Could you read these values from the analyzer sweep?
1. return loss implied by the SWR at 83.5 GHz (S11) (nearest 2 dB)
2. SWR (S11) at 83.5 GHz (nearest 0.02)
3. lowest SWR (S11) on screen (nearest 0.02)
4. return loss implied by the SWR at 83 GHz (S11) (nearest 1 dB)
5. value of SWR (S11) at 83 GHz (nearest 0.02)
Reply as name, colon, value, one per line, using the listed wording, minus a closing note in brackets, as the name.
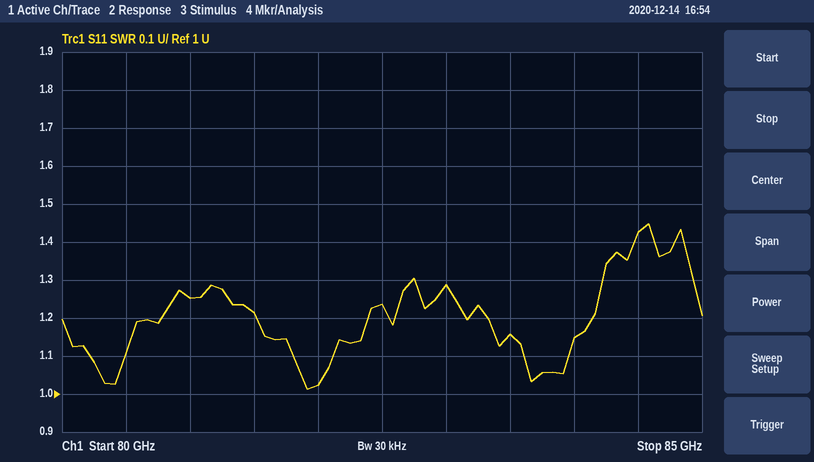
return loss implied by the SWR at 83.5 GHz (S11): 22 dB
SWR (S11) at 83.5 GHz: 1.16
lowest SWR (S11) on screen: 1.02
return loss implied by the SWR at 83 GHz (S11): 18 dB
value of SWR (S11) at 83 GHz: 1.28
